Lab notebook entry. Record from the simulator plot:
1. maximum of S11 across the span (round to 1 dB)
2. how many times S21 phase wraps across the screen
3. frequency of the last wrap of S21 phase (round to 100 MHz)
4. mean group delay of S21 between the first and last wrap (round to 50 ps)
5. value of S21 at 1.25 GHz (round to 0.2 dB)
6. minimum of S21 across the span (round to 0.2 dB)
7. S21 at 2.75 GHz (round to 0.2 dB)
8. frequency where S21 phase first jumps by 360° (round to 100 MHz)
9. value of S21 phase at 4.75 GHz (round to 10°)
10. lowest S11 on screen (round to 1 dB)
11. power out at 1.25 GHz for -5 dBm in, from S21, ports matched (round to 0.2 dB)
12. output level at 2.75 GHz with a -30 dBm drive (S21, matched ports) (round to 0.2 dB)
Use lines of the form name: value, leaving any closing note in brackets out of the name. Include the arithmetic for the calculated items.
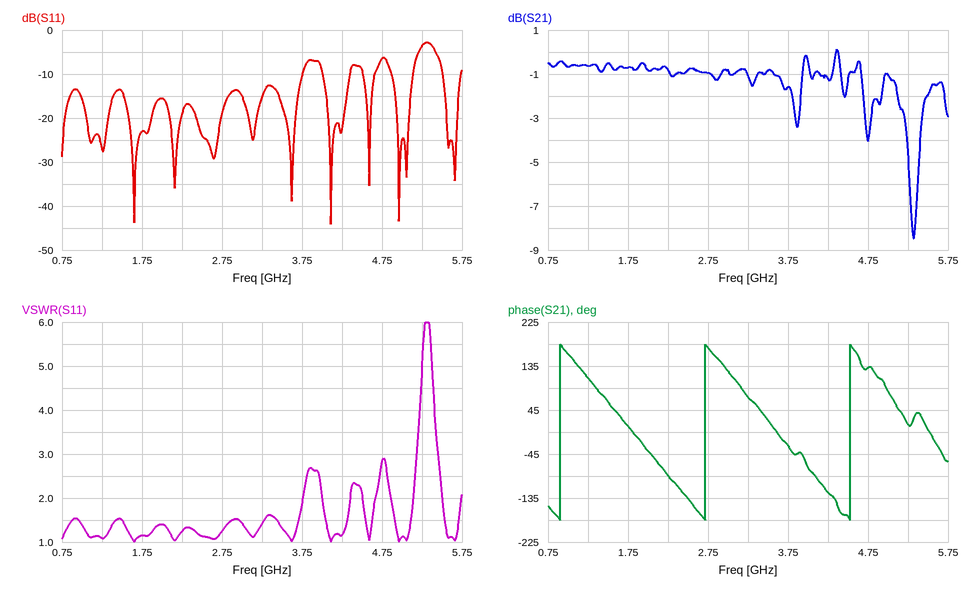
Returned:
maximum of S11 across the span: -3 dB
how many times S21 phase wraps across the screen: 3
frequency of the last wrap of S21 phase: 4.5 GHz
mean group delay of S21 between the first and last wrap: 2 cycles / (4.5 GHz − 900 MHz) ≈ 556 ps, so 550 ps to the nearest 50 ps
value of S21 at 1.25 GHz: -0.6 dB
minimum of S21 across the span: -8.4 dB
S21 at 2.75 GHz: -1.0 dB
frequency where S21 phase first jumps by 360°: 900 MHz
value of S21 phase at 4.75 GHz: 130°
lowest S11 on screen: -44 dB
power out at 1.25 GHz for -5 dBm in, from S21, ports matched: -5 dBm + (-0.6 dB) = -5.6 dBm
output level at 2.75 GHz with a -30 dBm drive (S21, matched ports): -30 dBm + (-1.0 dB) = -31.0 dBm
